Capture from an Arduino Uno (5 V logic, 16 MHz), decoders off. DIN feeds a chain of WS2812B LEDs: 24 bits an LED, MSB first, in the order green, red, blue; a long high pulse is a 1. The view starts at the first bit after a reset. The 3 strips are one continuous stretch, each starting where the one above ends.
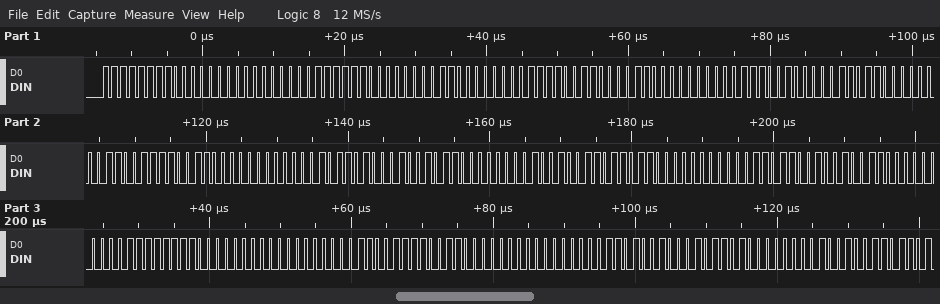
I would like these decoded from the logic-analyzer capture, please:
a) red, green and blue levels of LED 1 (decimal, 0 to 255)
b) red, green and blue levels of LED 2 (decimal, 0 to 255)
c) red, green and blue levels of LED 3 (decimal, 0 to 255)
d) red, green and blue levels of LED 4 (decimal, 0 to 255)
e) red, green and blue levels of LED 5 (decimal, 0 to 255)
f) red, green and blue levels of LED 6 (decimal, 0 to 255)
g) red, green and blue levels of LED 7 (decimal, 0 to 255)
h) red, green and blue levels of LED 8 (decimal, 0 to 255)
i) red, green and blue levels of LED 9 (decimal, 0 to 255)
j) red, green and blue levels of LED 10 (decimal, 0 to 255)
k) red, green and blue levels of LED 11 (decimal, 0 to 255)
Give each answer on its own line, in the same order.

0, 255, 0
3, 252, 0
12, 243, 0
27, 228, 0
48, 207, 0
75, 180, 0
108, 147, 0
147, 108, 0
192, 63, 0
243, 12, 0
210, 0, 45
